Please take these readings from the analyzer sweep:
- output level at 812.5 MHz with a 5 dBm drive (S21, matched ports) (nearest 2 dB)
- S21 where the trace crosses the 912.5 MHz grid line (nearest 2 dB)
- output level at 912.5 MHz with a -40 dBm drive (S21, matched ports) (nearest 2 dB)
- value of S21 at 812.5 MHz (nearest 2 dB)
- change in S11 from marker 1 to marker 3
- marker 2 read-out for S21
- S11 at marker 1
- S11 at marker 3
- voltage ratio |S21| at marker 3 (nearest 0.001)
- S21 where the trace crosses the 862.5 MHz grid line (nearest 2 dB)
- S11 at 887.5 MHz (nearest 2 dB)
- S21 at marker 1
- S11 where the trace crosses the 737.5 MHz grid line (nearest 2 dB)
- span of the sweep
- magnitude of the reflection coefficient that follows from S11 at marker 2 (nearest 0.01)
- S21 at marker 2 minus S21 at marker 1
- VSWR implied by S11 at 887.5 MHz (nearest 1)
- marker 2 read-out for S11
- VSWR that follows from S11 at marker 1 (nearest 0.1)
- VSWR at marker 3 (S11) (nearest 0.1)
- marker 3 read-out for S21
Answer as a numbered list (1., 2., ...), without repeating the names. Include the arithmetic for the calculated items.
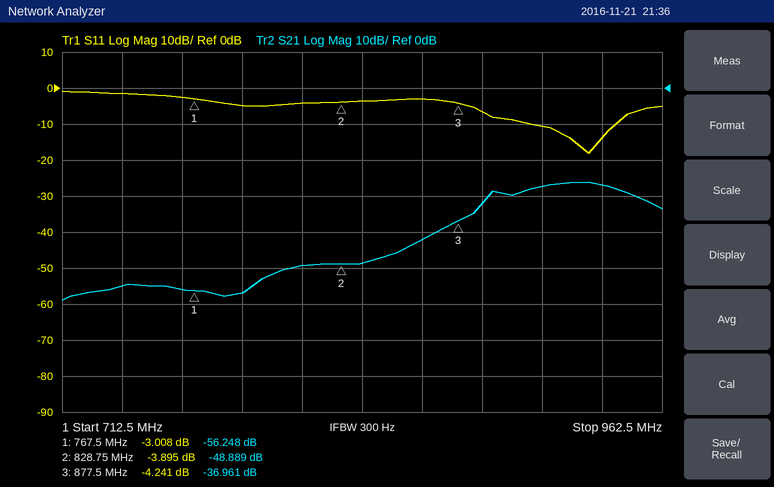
1. 5 dBm + (-50 dB) = -44 dBm
2. -28 dB
3. -40 dBm + (-28 dB) = -68 dBm
4. -50 dB
5. -4.241 − (-3.008) = -1.233 dB
6. -48.889 dB
7. -3.008 dB
8. -4.241 dB
9. 10^(-36.961/20) ≈ 0.014
10. -42 dB
11. -6 dB
12. -56.248 dB
13. -2 dB
14. 250 MHz
15. 10^(-3.895/20) ≈ 0.64
16. -48.889 − (-56.248) = 7.359 dB
17. |Γ| = 10^(-6/20) = 0.5012; VSWR = (1 + 0.5012)/(1 − 0.5012) ≈ 3
18. -3.895 dB
19. (1 + 0.7073)/(1 − 0.7073) ≈ 5.8
20. (1 + 0.6137)/(1 − 0.6137) ≈ 4.2
21. -36.961 dB
